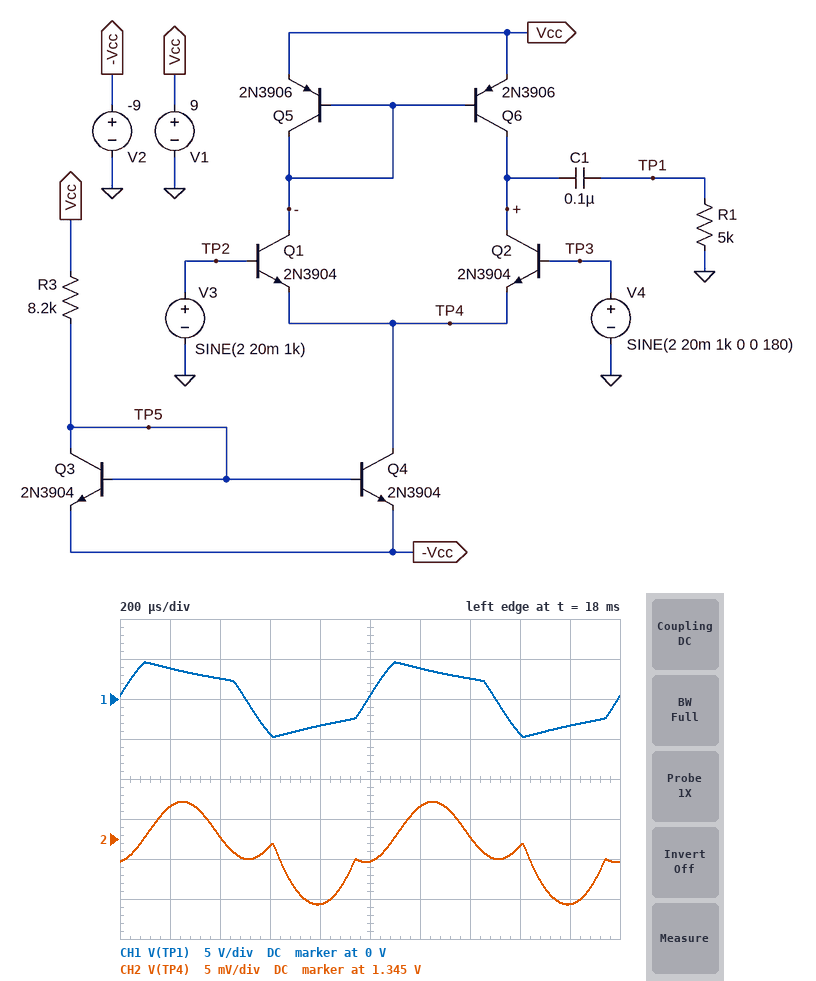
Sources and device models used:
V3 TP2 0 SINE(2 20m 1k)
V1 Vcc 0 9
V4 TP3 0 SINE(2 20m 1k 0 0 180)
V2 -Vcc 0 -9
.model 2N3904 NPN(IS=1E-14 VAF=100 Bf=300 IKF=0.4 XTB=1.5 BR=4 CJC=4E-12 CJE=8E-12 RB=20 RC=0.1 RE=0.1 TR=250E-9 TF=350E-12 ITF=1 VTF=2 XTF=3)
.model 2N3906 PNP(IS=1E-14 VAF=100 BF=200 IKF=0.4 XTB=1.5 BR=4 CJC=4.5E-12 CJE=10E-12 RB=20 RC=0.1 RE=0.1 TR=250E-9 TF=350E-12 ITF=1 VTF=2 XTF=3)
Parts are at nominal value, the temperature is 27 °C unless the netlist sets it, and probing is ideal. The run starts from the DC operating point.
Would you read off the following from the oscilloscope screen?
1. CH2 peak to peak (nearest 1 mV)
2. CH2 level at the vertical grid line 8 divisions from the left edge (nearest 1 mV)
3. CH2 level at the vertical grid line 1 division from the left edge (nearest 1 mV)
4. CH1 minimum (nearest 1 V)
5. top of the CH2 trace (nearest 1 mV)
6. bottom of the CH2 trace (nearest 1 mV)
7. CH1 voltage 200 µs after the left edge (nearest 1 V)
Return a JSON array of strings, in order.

["13 mV", "1.344 V", "1.349 V", "-5 V", "1.350 V", "1.337 V", "4 V"]
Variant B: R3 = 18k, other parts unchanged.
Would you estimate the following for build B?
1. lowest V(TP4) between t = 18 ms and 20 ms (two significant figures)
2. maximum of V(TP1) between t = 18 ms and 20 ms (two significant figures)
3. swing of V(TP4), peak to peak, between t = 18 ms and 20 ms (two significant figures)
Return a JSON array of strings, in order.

["1.4 V", "3.2 V", "7.5 mV"]
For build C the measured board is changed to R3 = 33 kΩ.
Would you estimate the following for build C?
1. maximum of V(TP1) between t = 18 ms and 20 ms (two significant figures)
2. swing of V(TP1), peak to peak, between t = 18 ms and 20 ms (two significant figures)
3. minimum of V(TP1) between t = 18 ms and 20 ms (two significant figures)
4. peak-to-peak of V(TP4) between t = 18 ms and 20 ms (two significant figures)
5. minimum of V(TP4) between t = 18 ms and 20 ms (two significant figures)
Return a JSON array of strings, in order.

["1.8 V", "3.6 V", "-1.8 V", "7.3 mV", "1.4 V"]
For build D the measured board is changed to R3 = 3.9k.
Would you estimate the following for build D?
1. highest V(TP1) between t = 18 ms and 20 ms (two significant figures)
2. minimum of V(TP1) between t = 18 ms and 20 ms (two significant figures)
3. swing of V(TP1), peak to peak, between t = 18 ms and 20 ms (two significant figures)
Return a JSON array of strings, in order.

["5.0 V", "-5.1 V", "10 V"]
